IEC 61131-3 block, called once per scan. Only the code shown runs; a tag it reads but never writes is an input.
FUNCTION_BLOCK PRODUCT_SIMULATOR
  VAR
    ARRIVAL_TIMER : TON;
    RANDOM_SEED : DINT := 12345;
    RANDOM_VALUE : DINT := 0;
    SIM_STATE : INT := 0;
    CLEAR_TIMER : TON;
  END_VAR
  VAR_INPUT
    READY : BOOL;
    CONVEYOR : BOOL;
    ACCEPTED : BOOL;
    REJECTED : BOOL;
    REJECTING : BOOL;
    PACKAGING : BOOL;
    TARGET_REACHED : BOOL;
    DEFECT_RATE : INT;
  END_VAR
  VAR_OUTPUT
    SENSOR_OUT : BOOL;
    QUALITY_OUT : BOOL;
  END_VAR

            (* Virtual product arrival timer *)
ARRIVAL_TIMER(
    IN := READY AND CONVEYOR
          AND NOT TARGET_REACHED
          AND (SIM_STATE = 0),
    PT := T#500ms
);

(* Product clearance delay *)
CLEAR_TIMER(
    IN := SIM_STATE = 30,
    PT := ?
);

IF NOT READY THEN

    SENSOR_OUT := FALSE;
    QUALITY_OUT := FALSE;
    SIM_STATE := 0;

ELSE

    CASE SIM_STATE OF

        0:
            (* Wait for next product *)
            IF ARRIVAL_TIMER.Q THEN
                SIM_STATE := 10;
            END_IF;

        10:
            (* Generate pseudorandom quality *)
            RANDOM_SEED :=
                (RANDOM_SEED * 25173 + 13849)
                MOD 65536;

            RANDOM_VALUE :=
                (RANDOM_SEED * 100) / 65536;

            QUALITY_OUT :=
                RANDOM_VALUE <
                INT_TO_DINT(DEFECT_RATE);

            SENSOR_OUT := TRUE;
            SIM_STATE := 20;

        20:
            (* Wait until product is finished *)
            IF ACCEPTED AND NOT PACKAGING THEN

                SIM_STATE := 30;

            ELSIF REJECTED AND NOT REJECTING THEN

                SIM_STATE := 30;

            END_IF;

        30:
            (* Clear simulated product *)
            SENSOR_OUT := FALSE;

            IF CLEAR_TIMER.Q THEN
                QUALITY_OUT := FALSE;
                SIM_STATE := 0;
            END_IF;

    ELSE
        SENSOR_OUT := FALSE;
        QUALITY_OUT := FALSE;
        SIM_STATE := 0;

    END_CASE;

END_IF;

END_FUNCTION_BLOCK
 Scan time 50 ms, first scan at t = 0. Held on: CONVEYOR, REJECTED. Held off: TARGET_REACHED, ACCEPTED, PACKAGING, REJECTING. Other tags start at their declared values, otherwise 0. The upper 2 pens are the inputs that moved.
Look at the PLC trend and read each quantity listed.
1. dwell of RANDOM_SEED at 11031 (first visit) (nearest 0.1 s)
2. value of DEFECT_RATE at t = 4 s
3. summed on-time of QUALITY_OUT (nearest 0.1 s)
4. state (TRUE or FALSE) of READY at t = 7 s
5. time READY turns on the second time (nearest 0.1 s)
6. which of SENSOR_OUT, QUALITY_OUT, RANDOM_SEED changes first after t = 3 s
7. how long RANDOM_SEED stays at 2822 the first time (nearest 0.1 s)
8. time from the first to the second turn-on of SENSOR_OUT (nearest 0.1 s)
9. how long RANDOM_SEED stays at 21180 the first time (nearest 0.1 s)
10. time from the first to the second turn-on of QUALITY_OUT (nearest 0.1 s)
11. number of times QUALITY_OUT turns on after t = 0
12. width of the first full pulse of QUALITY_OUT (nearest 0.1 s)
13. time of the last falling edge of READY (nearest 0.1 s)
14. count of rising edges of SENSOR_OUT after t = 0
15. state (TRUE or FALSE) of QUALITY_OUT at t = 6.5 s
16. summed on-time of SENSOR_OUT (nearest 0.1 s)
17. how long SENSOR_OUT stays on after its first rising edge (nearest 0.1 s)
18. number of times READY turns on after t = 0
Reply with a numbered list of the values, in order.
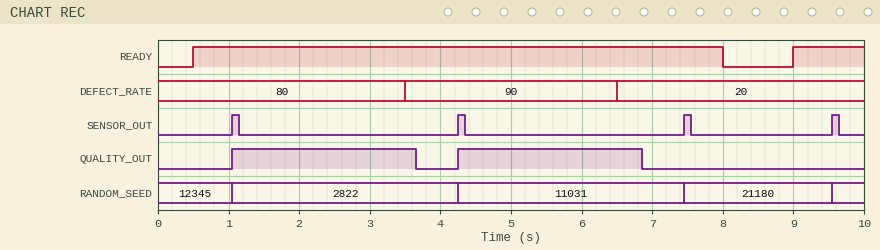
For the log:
1. 3.2 s
2. 90
3. 5.2 s
4. TRUE
5. 9.0 s
6. QUALITY_OUT
7. 3.2 s
8. 3.2 s
9. 2.1 s
10. 3.2 s
11. 2
12. 2.6 s
13. 8.0 s
14. 4
15. TRUE
16. 0.4 s
17. 0.1 s
18. 2
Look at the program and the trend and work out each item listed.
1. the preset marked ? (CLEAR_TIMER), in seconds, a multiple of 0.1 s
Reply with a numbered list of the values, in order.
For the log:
1. 2.5 s
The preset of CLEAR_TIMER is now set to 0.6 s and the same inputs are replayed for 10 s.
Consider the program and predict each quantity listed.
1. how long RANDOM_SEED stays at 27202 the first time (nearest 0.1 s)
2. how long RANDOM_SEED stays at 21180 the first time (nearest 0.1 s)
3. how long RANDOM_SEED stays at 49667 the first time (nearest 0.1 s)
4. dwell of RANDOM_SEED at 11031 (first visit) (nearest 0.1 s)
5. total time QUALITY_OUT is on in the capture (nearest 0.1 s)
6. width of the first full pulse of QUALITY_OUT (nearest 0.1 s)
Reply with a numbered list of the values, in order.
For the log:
1. 1.3 s
2. 1.3 s
3. 2.0 s
4. 1.3 s
5. 3.5 s
6. 0.7 s
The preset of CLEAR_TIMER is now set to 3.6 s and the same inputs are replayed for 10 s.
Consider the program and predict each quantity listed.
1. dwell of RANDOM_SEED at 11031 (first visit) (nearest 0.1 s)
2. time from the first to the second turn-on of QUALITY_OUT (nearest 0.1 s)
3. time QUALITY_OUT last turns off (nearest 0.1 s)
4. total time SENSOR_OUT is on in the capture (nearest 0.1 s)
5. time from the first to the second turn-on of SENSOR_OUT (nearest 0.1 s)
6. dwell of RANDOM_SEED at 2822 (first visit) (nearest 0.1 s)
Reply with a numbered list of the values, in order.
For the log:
1. 4.2 s
2. 4.3 s
3. 8.0 s
4. 0.3 s
5. 4.3 s
6. 4.3 s
